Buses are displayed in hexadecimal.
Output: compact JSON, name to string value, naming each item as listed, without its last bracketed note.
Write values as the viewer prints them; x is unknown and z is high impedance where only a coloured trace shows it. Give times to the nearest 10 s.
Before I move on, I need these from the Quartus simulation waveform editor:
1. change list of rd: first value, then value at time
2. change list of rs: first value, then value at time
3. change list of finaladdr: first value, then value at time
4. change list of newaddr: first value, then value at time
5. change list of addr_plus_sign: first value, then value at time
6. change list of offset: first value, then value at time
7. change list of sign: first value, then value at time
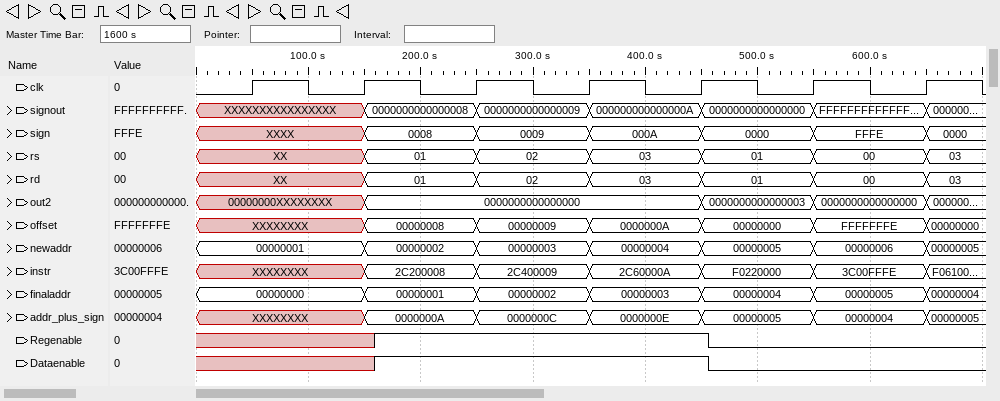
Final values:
{"change list of rd: first value, then value at time": "XX, 01 at 150 s, 02 at 250 s, 03 at 350 s, 01 at 450 s, 00 at 550 s, 03 at 650 s", "change list of rs: first value, then value at time": "XX, 01 at 150 s, 02 at 250 s, 03 at 350 s, 01 at 450 s, 00 at 550 s, 03 at 650 s", "change list of finaladdr: first value, then value at time": "00000000, 00000001 at 150 s, 00000002 at 250 s, 00000003 at 350 s, 00000004 at 450 s, 00000005 at 550 s, 00000004 at 650 s", "change list of newaddr: first value, then value at time": "00000001, 00000002 at 150 s, 00000003 at 250 s, 00000004 at 350 s, 00000005 at 450 s, 00000006 at 550 s, 00000005 at 650 s", "change list of addr_plus_sign: first value, then value at time": "XXXXXXXX, 0000000A at 150 s, 0000000C at 250 s, 0000000E at 350 s, 00000005 at 450 s, 00000004 at 550 s, 00000005 at 650 s", "change list of offset: first value, then value at time": "XXXXXXXX, 00000008 at 150 s, 00000009 at 250 s, 0000000A at 350 s, 00000000 at 450 s, FFFFFFFE at 550 s, 00000000 at 650 s", "change list of sign: first value, then value at time": "XXXX, 0008 at 150 s, 0009 at 250 s, 000A at 350 s, 0000 at 450 s, FFFE at 550 s, 0000 at 650 s"}
